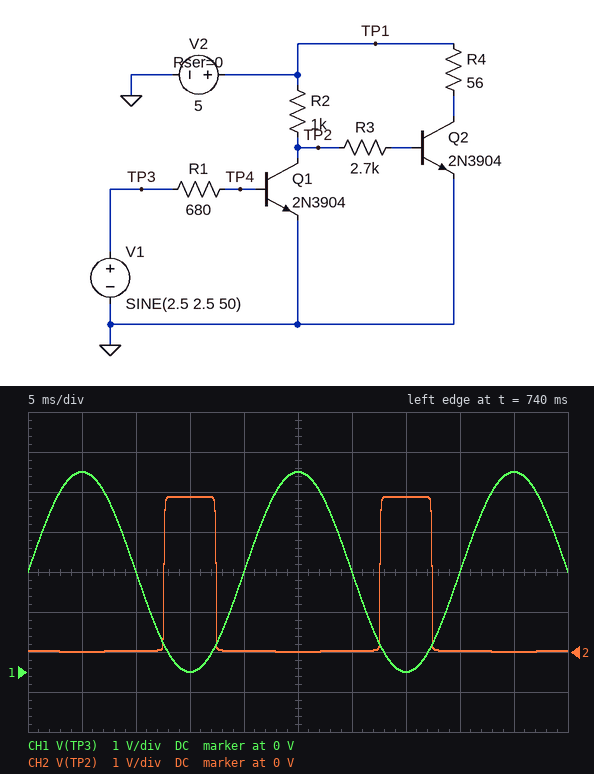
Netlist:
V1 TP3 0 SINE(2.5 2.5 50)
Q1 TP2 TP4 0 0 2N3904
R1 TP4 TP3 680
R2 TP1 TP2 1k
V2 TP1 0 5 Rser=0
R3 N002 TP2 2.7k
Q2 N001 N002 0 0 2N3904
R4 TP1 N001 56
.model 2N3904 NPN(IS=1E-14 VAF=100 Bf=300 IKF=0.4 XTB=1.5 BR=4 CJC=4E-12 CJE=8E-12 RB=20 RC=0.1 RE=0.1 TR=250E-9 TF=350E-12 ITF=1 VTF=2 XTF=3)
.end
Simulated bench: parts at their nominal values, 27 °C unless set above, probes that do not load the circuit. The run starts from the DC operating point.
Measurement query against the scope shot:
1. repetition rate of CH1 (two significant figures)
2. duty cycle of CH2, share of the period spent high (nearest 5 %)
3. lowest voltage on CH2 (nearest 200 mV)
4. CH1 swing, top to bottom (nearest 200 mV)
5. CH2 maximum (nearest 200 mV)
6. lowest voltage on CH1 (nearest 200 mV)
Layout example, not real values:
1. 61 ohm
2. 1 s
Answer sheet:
1. 50 Hz
2. 25 %
3. 0 V
4. 5.0 V
5. 3.8 V
6. 0 V
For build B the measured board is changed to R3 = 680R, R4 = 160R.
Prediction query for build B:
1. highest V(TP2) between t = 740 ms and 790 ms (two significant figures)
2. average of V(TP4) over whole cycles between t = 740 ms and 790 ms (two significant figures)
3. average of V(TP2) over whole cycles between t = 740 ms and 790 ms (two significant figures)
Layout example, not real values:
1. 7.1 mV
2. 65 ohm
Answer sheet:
1. 2.5 V
2. 670 mV
3. 620 mV
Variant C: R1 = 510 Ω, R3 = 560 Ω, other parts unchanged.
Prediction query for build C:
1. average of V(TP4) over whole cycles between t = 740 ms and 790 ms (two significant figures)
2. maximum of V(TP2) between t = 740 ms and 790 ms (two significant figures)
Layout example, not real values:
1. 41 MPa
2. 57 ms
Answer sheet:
1. 690 mV
2. 2.3 V
